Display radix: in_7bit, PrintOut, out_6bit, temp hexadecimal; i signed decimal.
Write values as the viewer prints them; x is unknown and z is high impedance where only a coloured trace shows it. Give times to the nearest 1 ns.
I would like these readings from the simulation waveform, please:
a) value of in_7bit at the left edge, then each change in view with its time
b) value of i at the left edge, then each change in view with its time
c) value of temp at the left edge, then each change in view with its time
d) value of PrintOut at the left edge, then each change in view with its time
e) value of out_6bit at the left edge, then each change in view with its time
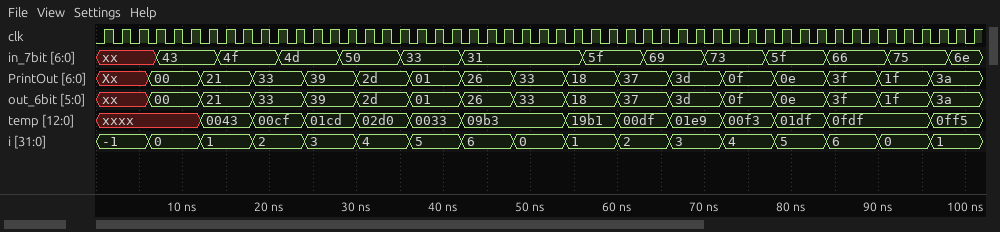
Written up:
xx, 43 at 7 ns, 4f at 14 ns, 4d at 21 ns, 50 at 28 ns, 33 at 35 ns, 31 at 42 ns, 5f at 56 ns, 69 at 63 ns, 73 at 70 ns, 5f at 77 ns, 66 at 84 ns, 75 at 91 ns, 6e at 98 ns
-1, 0 at 6 ns, 1 at 12 ns, 2 at 18 ns, 3 at 24 ns, 4 at 30 ns, 5 at 36 ns, 6 at 42 ns, 0 at 48 ns, 1 at 54 ns, 2 at 60 ns, 3 at 66 ns, 4 at 72 ns, 5 at 78 ns, 6 at 84 ns, 0 at 90 ns, 1 at 96 ns
xxxx, 0043 at 12 ns, 00cf at 18 ns, 01cd at 24 ns, 02d0 at 30 ns, 0033 at 36 ns, 09b3 at 42 ns, 19b1 at 54 ns, 00df at 60 ns, 01e9 at 66 ns, 00f3 at 72 ns, 01df at 78 ns, 0fdf at 84 ns, 0ff5 at 96 ns
Xx, 00 at 6 ns, 21 at 12 ns, 33 at 18 ns, 39 at 24 ns, 2d at 30 ns, 01 at 36 ns, 26 at 42 ns, 33 at 48 ns, 18 at 54 ns, 37 at 60 ns, 3d at 66 ns, 0f at 72 ns, 0e at 78 ns, 3f at 84 ns, 1f at 90 ns, 3a at 96 ns
xx, 00 at 6 ns, 21 at 12 ns, 33 at 18 ns, 39 at 24 ns, 2d at 30 ns, 01 at 36 ns, 26 at 42 ns, 33 at 48 ns, 18 at 54 ns, 37 at 60 ns, 3d at 66 ns, 0f at 72 ns, 0e at 78 ns, 3f at 84 ns, 1f at 90 ns, 3a at 96 ns
